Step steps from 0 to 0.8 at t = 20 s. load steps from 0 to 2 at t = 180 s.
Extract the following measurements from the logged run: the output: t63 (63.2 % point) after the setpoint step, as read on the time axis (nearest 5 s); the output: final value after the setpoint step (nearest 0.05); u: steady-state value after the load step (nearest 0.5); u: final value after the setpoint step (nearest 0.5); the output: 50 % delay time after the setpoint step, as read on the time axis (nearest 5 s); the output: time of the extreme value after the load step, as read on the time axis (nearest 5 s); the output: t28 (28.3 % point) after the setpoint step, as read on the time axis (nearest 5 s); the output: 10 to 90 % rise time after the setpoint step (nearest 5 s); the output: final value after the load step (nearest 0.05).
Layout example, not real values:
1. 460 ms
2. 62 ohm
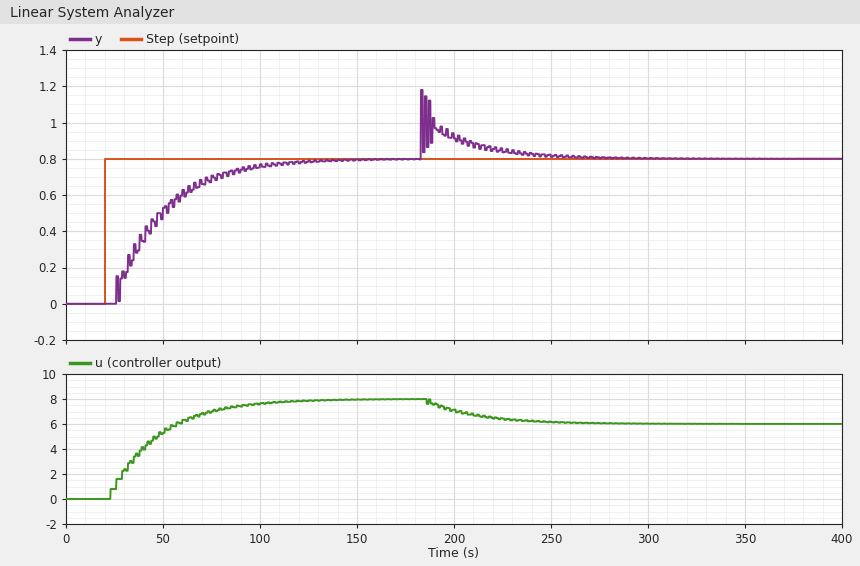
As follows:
1. 50 s
2. 0.80
3. 6.0
4. 8.0
5. 40 s
6. 185 s
7. 30 s
8. 55 s
9. 0.80
